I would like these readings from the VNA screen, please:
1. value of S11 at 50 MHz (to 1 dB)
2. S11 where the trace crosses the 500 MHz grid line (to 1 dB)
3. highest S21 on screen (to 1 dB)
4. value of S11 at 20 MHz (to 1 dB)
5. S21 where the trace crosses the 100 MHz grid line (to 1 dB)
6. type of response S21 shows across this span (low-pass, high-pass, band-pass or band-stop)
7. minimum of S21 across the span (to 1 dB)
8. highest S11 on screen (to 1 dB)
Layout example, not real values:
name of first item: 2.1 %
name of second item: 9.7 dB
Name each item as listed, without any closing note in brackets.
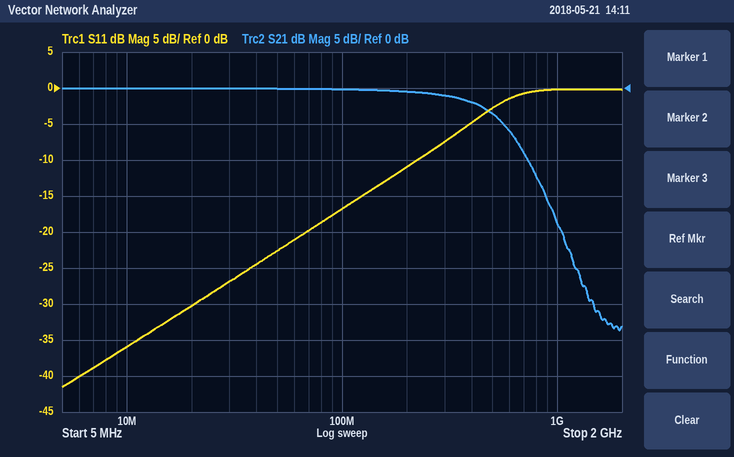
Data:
value of S11 at 50 MHz: -23 dB
S11 where the trace crosses the 500 MHz grid line: -3 dB
highest S21 on screen: 0 dB
value of S11 at 20 MHz: -30 dB
S21 where the trace crosses the 100 MHz grid line: 0 dB
type of response S21 shows across this span: low-pass
minimum of S21 across the span: -34 dB
highest S11 on screen: 0 dB
